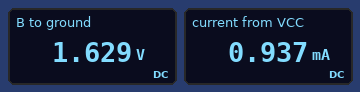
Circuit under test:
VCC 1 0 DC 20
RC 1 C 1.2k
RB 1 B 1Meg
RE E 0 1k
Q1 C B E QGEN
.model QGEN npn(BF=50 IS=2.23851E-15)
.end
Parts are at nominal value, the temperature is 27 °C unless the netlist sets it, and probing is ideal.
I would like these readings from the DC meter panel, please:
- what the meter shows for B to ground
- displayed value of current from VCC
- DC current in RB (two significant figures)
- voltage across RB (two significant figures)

1.629 V
0.937 mA
18 µA
18 V
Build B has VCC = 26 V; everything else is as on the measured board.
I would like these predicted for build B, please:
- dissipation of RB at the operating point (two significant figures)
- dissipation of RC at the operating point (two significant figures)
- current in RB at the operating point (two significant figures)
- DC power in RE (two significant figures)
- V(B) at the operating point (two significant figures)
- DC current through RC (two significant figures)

580 µW
1.7 mW
24 µA
1.5 mW
1.9 V
1.2 mA
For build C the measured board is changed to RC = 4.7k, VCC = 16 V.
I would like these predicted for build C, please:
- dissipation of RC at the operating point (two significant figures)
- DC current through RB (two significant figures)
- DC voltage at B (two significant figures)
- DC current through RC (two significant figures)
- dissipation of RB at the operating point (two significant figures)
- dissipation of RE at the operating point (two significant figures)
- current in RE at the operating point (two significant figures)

2.5 mW
15 µA
1.4 V
730 µA
210 µW
550 µW
740 µA
